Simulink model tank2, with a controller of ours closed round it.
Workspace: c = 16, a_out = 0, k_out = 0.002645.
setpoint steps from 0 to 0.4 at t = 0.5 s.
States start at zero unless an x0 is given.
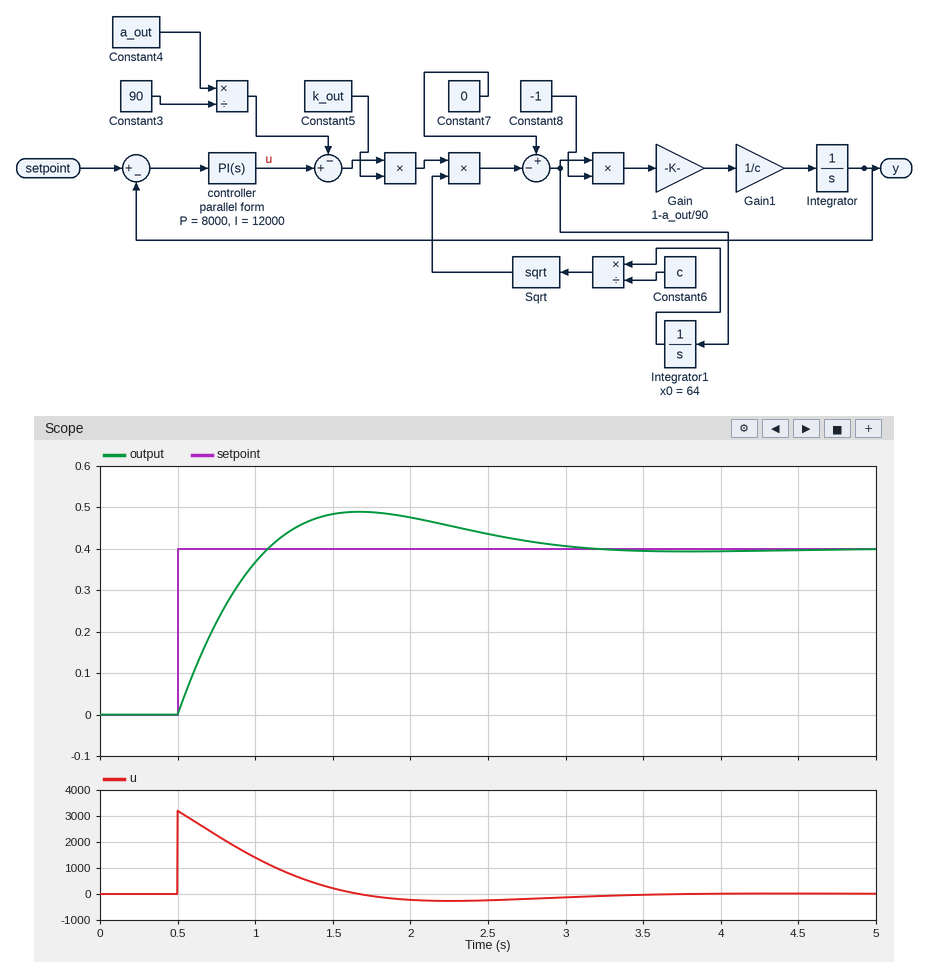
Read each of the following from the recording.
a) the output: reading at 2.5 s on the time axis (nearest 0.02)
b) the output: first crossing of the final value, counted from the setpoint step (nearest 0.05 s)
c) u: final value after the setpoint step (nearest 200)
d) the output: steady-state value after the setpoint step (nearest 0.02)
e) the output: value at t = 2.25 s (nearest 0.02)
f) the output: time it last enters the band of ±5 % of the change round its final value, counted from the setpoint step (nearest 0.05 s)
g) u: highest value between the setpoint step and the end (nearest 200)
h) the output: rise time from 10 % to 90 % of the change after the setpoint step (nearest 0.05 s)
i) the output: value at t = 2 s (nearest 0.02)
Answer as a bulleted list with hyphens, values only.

- 0.44
- 0.60 s
- 0
- 0.40
- 0.46
- 2.25 s
- 3200
- 0.45 s
- 0.48
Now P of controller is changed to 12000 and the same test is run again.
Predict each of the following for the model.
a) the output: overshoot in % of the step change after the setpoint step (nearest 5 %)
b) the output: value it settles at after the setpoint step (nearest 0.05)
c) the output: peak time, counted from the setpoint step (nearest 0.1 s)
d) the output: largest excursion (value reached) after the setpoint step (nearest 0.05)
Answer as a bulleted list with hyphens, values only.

- 15 %
- 0.40
- 1.0 s
- 0.45
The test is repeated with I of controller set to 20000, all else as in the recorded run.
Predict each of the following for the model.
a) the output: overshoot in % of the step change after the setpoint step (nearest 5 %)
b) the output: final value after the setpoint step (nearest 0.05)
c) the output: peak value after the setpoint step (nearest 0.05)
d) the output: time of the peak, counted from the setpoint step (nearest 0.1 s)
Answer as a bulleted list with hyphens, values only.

- 30 %
- 0.40
- 0.50
- 1.0 s
